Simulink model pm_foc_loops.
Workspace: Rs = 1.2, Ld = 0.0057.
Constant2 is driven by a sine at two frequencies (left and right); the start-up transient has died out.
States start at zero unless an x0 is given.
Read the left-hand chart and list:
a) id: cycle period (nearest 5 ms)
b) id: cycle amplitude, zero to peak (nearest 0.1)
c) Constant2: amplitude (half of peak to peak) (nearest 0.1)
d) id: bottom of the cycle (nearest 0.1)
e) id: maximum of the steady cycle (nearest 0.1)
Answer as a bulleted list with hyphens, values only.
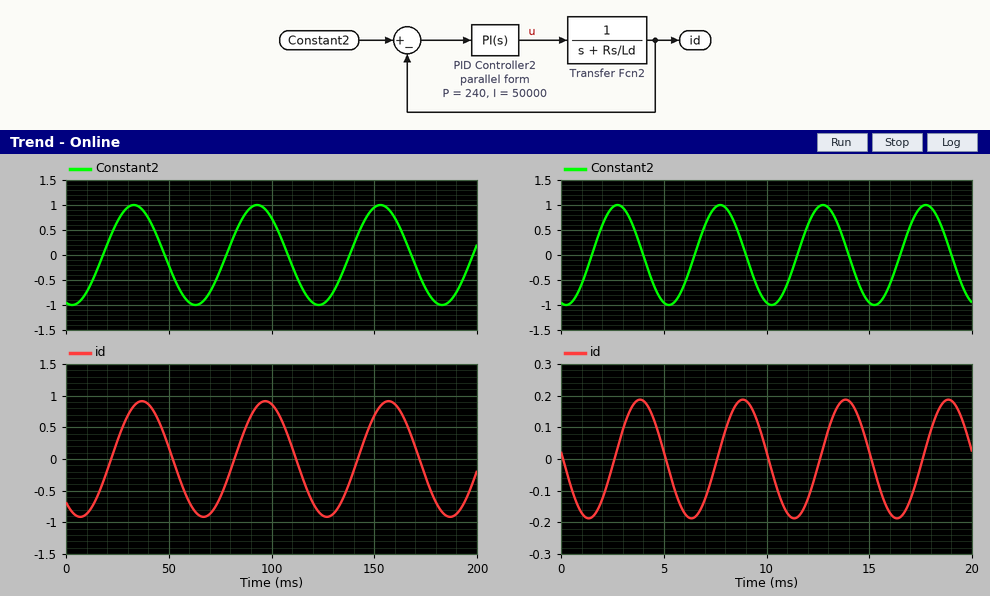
- 60 ms
- 0.9
- 1.0
- -0.9
- 0.9
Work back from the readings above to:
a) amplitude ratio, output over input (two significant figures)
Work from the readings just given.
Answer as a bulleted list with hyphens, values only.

- 0.90
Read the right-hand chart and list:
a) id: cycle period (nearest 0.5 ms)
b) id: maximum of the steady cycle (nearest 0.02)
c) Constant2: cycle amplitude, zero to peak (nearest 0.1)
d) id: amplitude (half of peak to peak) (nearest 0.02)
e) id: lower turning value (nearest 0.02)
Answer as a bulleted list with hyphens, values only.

- 5.0 ms
- 0.18
- 1.0
- 0.18
- -0.18
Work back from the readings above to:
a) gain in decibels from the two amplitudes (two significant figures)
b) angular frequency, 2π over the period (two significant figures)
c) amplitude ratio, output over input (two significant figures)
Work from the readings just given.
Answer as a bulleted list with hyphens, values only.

- -15 dB
- 1.3 rad/ms
- 0.18
